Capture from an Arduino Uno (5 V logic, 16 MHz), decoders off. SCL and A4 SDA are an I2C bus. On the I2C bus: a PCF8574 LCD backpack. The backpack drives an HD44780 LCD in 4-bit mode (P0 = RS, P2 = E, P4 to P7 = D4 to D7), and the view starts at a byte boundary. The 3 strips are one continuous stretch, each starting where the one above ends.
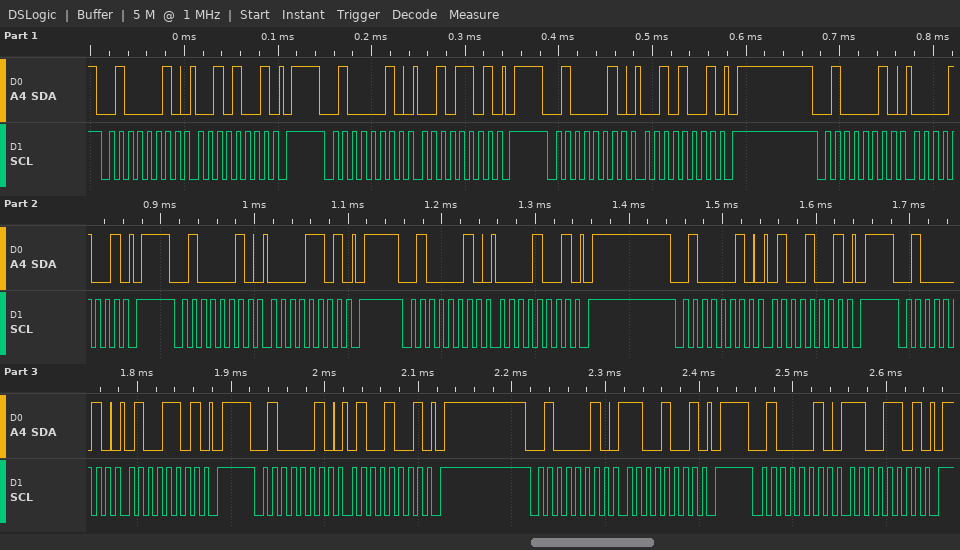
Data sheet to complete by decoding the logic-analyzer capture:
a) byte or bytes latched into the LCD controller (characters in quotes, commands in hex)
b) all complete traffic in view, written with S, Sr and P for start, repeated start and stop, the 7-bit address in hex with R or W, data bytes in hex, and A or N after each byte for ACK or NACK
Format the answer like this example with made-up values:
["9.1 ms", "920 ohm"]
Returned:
["' '", "S 21W A 29 A P S 21W A 2D A P S 21W A 29 A P S 21W A 09 A P S 21W A 0D A P S 21W A 09 A P S 21W A 49 A P S 21W A 4D A P S 21W A 49 A P S 21W A C9 A P S 21W A CD A P"]
